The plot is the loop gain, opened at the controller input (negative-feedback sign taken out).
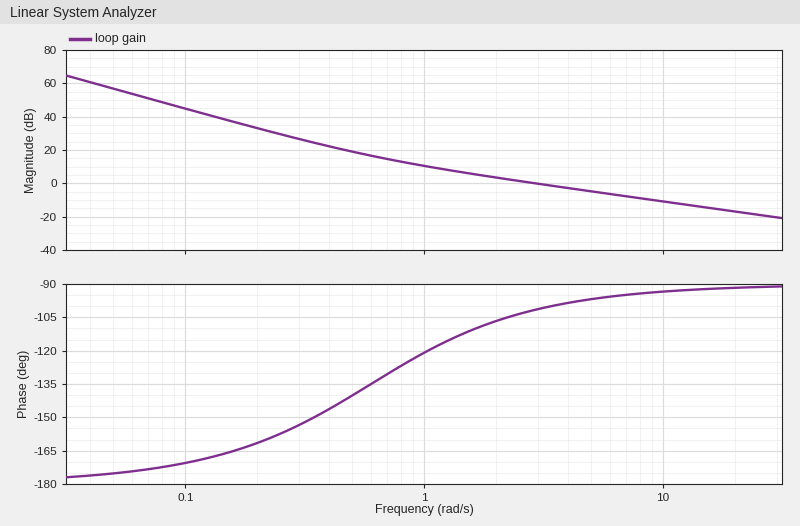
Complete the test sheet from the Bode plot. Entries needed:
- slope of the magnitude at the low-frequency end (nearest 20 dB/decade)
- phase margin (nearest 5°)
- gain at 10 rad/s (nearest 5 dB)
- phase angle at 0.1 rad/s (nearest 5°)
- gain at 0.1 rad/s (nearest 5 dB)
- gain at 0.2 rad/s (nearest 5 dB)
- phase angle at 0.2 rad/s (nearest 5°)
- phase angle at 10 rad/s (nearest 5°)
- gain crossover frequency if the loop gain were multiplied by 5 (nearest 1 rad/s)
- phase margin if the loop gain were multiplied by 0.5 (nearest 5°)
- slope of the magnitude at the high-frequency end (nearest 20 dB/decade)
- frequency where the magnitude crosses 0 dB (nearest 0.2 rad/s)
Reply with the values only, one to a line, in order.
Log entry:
-40 dB/decade
80°
-10 dB
-170°
45 dB
35 dB
-160°
-95°
14 rad/s
70°
-20 dB/decade
3.0 rad/s
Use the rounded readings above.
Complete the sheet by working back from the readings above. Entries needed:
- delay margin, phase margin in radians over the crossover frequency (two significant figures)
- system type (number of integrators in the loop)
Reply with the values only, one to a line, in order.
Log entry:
0.47 s
2
